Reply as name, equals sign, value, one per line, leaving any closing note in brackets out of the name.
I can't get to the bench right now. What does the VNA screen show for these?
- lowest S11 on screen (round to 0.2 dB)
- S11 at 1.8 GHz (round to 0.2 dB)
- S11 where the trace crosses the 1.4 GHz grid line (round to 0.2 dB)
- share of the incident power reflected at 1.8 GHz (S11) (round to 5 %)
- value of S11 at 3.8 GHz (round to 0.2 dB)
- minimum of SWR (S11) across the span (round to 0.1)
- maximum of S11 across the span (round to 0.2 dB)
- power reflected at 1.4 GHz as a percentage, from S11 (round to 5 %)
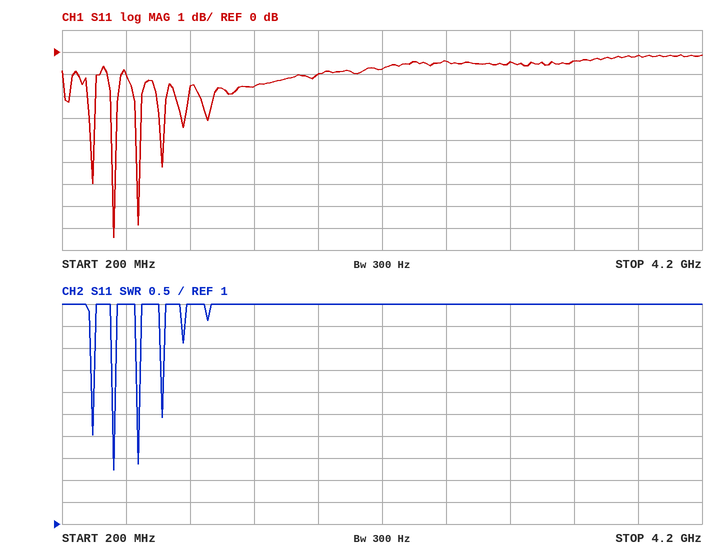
lowest S11 on screen = -8.4 dB
S11 at 1.8 GHz = -1.0 dB
S11 where the trace crosses the 1.4 GHz grid line = -1.6 dB
share of the incident power reflected at 1.8 GHz (S11) = 80 %
value of S11 at 3.8 GHz = -0.2 dB
minimum of SWR (S11) across the span = 2.2
maximum of S11 across the span = -0.2 dB
power reflected at 1.4 GHz as a percentage, from S11 = 70 %
